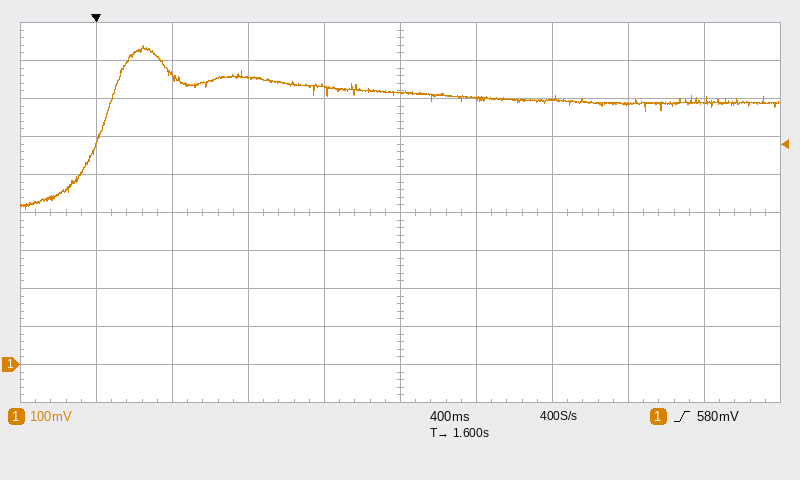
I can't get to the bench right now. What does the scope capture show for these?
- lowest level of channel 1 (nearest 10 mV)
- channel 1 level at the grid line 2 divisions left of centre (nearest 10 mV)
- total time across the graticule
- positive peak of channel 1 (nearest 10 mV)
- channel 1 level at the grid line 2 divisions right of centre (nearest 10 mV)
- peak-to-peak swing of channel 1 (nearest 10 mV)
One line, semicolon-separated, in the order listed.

410 mV; 750 mV; 4 s; 840 mV; 700 mV; 430 mV
